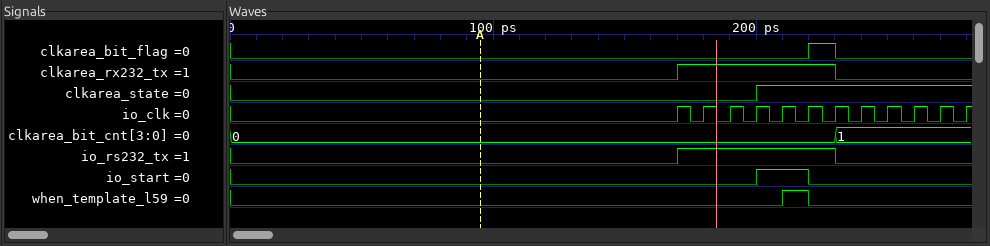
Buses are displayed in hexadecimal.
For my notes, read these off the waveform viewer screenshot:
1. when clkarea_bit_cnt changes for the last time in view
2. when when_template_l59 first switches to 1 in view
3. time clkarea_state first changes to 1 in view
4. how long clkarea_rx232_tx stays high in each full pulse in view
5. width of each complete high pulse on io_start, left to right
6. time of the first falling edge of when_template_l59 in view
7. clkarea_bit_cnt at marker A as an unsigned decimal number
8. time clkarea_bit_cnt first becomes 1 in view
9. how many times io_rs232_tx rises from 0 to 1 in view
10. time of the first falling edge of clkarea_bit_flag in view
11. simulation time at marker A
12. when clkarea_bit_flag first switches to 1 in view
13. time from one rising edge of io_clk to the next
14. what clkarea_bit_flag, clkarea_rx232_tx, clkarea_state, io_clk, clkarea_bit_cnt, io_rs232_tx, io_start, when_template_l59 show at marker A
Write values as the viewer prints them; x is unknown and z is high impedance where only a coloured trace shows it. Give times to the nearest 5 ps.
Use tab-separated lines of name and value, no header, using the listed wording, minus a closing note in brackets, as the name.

when clkarea_bit_cnt changes for the last time in view	230 ps
when when_template_l59 first switches to 1 in view	210 ps
time clkarea_state first changes to 1 in view	200 ps
how long clkarea_rx232_tx stays high in each full pulse in view	60 ps
width of each complete high pulse on io_start, left to right	20 ps
time of the first falling edge of when_template_l59 in view	220 ps
clkarea_bit_cnt at marker A as an unsigned decimal number	0
time clkarea_bit_cnt first becomes 1 in view	230 ps
how many times io_rs232_tx rises from 0 to 1 in view	1
time of the first falling edge of clkarea_bit_flag in view	230 ps
simulation time at marker A	95 ps
when clkarea_bit_flag first switches to 1 in view	220 ps
time from one rising edge of io_clk to the next	10 ps
what clkarea_bit_flag, clkarea_rx232_tx, clkarea_state, io_clk, clkarea_bit_cnt, io_rs232_tx, io_start, when_template_l59 show at marker A	clkarea_bit_flag=0, clkarea_rx232_tx=0, clkarea_state=0, io_clk=0, clkarea_bit_cnt=0, io_rs232_tx=0, io_start=0, when_template_l59=0
